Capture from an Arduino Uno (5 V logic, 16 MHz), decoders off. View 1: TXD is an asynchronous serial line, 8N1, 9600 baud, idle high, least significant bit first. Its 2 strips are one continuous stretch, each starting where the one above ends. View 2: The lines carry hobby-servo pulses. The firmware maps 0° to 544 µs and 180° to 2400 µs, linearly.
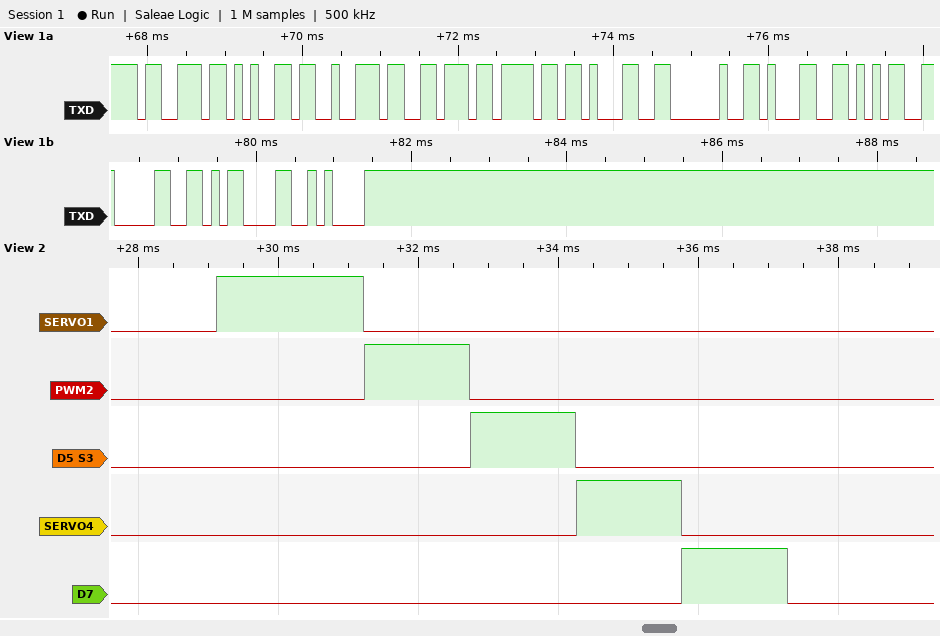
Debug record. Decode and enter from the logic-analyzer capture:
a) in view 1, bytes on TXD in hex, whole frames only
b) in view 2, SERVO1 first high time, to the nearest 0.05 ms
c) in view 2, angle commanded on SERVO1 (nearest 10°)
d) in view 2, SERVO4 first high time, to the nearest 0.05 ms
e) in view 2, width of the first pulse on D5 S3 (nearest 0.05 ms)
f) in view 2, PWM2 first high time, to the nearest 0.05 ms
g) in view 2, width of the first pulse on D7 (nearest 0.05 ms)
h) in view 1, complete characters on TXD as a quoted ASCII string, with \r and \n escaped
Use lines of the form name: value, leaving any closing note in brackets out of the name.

in view 1, bytes on TXD in hex, whole frames only: 73 65 72 76 6F 31 20 31 35 30 0D 0A
in view 2, SERVO1 first high time, to the nearest 0.05 ms: 2.10 ms
in view 2, angle commanded on SERVO1: 150°
in view 2, SERVO4 first high time, to the nearest 0.05 ms: 1.50 ms
in view 2, width of the first pulse on D5 S3: 1.50 ms
in view 2, PWM2 first high time, to the nearest 0.05 ms: 1.50 ms
in view 2, width of the first pulse on D7: 1.50 ms
in view 1, complete characters on TXD as a quoted ASCII string, with \r and \n escaped: "servo1 150\r\n"
